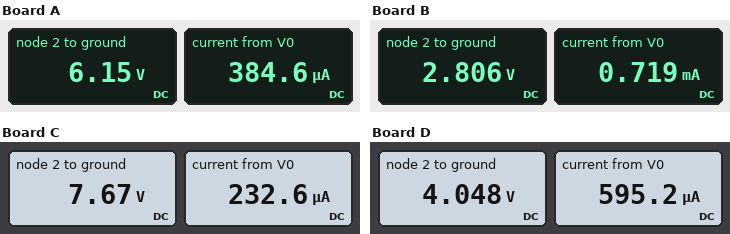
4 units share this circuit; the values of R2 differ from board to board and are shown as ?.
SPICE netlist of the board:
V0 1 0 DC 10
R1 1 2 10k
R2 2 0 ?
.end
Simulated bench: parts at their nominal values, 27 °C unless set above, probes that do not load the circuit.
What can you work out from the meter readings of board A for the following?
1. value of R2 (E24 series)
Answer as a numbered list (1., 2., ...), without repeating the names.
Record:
1. 16 kΩ
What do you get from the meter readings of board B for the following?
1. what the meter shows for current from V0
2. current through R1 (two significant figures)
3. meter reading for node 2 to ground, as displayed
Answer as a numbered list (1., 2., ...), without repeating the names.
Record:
1. 0.719 mA
2. 720 µA
3. 2.806 V
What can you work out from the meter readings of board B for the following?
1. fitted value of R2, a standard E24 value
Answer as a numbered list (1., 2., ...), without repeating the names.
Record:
1. 3.9 kΩ
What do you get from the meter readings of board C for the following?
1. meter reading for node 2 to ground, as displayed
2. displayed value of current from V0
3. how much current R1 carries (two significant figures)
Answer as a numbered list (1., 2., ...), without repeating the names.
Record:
1. 7.67 V
2. 232.6 µA
3. 230 µA
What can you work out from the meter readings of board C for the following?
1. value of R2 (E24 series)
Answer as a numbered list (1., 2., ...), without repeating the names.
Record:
1. 33 kΩ
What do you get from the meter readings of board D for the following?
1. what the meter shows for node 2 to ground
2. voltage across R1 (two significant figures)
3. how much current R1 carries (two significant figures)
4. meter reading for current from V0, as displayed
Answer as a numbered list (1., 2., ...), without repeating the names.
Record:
1. 4.048 V
2. 6.0 V
3. 600 µA
4. 595.2 µA
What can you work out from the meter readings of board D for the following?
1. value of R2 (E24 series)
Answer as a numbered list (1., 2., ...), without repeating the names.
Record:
1. 6.8 kΩ
